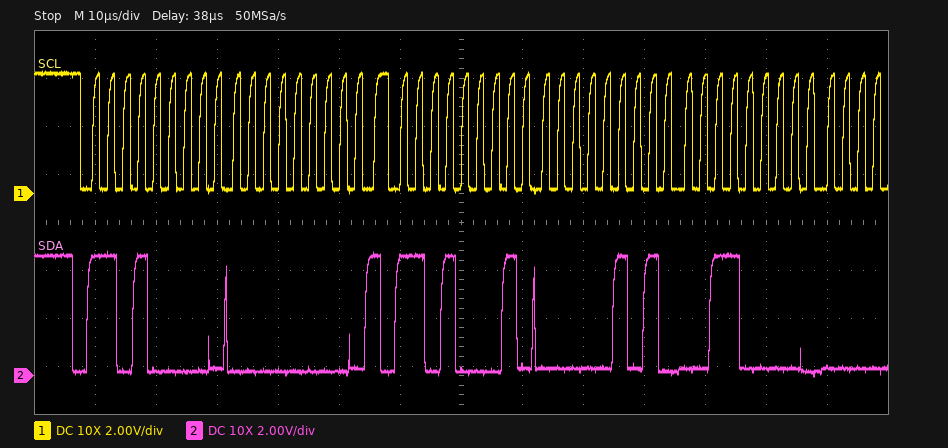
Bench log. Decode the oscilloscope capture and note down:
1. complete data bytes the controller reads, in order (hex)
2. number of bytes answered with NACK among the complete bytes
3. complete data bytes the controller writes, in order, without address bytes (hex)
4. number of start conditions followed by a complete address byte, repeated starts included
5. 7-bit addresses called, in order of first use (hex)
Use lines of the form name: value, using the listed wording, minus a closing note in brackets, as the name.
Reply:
complete data bytes the controller reads, in order: 05 30
number of bytes answered with NACK among the complete bytes: 0
complete data bytes the controller writes, in order, without address bytes: 00
number of start conditions followed by a complete address byte, repeated starts included: 2
7-bit addresses called, in order of first use: 0x68
